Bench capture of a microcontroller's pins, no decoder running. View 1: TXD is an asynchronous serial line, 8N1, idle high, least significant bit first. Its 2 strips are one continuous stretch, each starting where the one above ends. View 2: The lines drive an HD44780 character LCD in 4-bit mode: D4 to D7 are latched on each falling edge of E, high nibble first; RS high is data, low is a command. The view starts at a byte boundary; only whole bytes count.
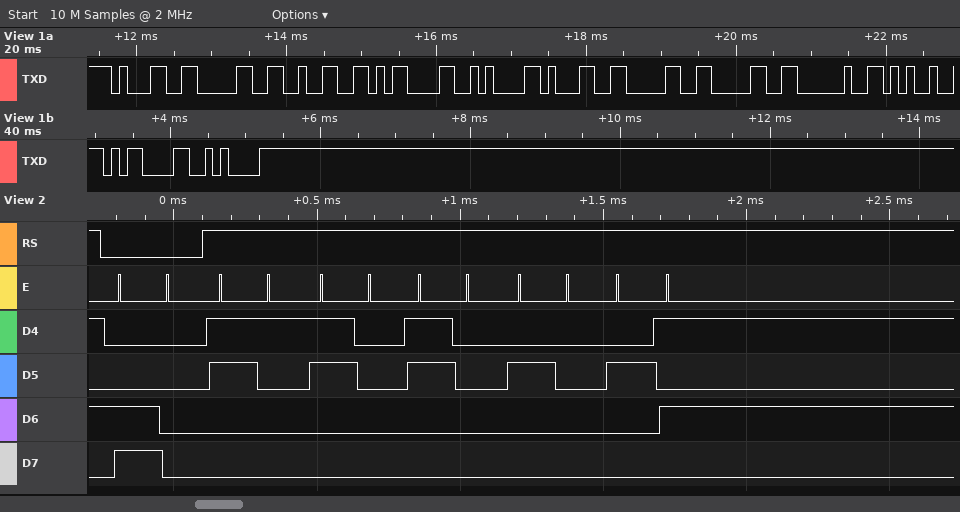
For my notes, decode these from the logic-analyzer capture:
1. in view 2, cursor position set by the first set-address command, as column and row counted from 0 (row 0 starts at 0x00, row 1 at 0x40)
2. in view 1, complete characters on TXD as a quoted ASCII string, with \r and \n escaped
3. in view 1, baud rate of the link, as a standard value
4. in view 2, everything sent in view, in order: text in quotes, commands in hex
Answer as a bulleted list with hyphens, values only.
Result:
- column 0, row 1
- "102\r\n100 %\r\n"
- 9600 baud
- 0xC0 "100 %"
